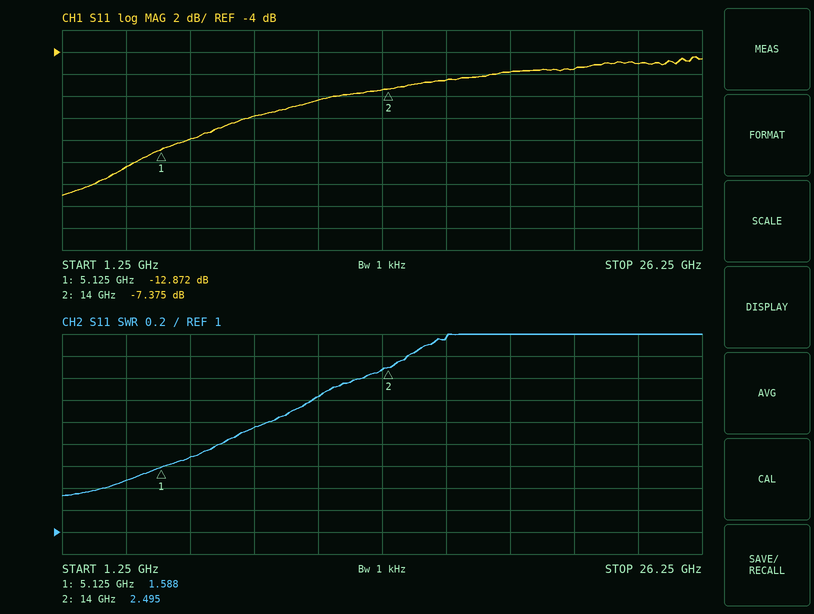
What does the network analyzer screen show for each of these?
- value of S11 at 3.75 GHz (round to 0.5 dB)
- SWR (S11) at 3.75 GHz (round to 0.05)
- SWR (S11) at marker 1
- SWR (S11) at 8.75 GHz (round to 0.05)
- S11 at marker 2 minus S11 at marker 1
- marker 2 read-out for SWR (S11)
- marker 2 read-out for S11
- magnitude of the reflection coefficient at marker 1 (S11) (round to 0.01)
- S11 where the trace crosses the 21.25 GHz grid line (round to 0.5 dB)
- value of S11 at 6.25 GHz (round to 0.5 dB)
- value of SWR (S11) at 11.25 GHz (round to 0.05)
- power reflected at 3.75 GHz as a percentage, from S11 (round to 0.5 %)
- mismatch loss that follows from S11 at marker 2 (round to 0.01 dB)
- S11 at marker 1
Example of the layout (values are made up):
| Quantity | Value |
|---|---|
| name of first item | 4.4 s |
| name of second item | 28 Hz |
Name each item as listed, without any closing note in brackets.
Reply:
| Quantity | Value |
|---|---|
| value of S11 at 3.75 GHz | -14.5 dB |
| SWR (S11) at 3.75 GHz | 1.45 |
| SWR (S11) at marker 1 | 1.588 |
| SWR (S11) at 8.75 GHz | 1.95 |
| S11 at marker 2 minus S11 at marker 1 | 5.497 dB |
| marker 2 read-out for SWR | 2.495 |
| marker 2 read-out for S11 | -7.375 dB |
| magnitude of the reflection coefficient at marker 1 (S11) | 0.23 |
| S11 where the trace crosses the 21.25 GHz grid line | -5.5 dB |
| value of S11 at 6.25 GHz | -12.0 dB |
| value of SWR (S11) at 11.25 GHz | 2.25 |
| power reflected at 3.75 GHz as a percentage, from S11 | 3.5 % |
| mismatch loss that follows from S11 at marker 2 | 0.88 dB |
| S11 at marker 1 | -12.872 dB |
